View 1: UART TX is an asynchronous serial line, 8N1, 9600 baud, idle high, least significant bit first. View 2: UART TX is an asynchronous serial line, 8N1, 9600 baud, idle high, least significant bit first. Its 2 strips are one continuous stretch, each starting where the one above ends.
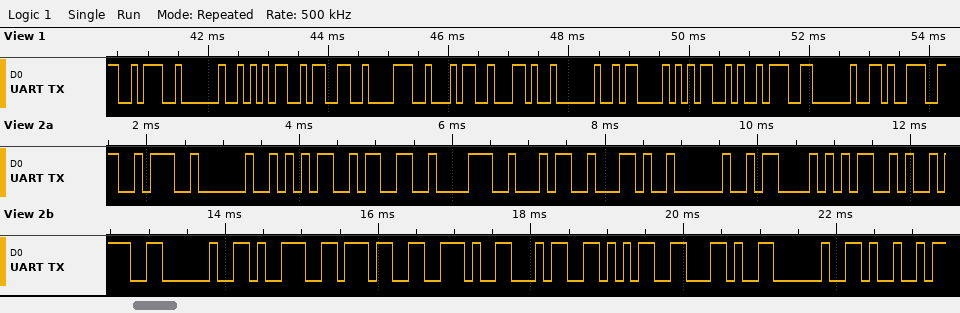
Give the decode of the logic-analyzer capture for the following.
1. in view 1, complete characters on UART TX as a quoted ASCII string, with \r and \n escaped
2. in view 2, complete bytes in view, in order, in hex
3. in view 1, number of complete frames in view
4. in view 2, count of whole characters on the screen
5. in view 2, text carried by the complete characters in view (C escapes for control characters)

": 5384, CM: 9"
0x3A 0x20 0x35 0x33 0x38 0x34 0x2C 0x20 0x43 0x4D 0x3A 0x20 0x39 0x37 0x2E 0x34 0x35 0x2C 0x20 0x49
13
20
": 5384, CM: 97.45, I"
